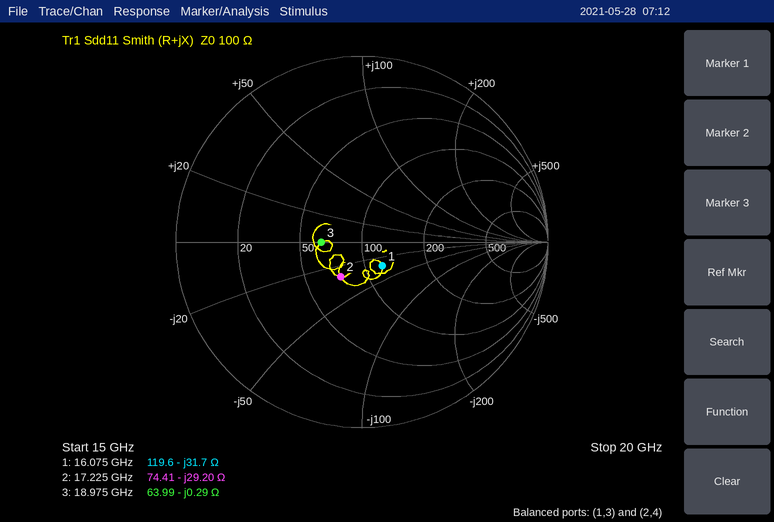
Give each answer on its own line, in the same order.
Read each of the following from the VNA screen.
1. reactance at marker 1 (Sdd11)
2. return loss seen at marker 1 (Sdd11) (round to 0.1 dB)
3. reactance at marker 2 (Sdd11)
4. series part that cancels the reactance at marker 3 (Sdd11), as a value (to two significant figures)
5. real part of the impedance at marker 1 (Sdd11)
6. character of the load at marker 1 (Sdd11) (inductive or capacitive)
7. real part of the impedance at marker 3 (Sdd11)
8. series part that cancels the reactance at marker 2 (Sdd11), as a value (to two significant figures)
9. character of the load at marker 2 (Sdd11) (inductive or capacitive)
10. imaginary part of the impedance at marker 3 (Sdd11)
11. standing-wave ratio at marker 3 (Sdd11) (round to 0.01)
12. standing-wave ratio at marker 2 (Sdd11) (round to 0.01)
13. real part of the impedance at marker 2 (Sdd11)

-31.7 Ω
15.5 dB
-29.20 Ω
2.4 pH
119.6 Ω
capacitive
63.99 Ω
270 pH
capacitive
-0.29 Ω
1.56
1.56
74.41 Ω
